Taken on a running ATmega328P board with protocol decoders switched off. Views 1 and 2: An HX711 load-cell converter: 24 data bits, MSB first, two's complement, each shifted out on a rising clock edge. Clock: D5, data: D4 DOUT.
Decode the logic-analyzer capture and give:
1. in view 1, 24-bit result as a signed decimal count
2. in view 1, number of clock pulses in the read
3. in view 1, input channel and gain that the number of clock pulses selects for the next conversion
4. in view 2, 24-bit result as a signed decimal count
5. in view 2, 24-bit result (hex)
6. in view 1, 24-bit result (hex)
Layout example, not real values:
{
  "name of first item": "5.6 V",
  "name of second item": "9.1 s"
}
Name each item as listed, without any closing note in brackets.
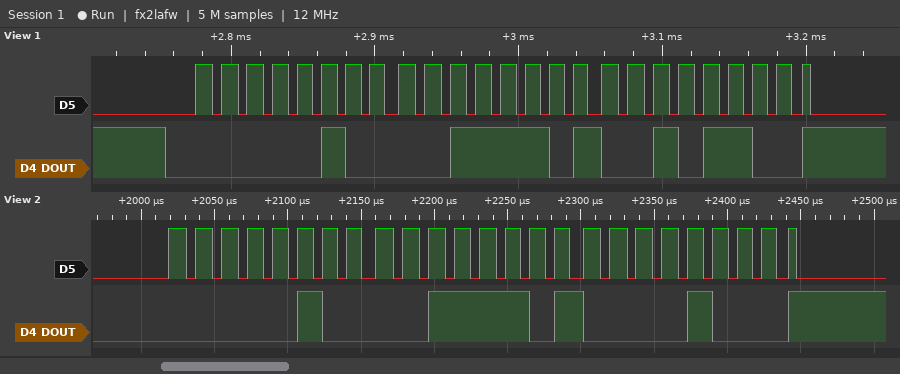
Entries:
{
  "in view 1, 24-bit result as a signed decimal count": "277804",
  "in view 1, number of clock pulses in the read": "25",
  "in view 1, input channel and gain that the number of clock pulses selects for the next conversion": "channel A, gain 128",
  "in view 2, 24-bit result as a signed decimal count": "277768",
  "in view 2, 24-bit result": "0x043D08",
  "in view 1, 24-bit result": "0x043D2C"
}
